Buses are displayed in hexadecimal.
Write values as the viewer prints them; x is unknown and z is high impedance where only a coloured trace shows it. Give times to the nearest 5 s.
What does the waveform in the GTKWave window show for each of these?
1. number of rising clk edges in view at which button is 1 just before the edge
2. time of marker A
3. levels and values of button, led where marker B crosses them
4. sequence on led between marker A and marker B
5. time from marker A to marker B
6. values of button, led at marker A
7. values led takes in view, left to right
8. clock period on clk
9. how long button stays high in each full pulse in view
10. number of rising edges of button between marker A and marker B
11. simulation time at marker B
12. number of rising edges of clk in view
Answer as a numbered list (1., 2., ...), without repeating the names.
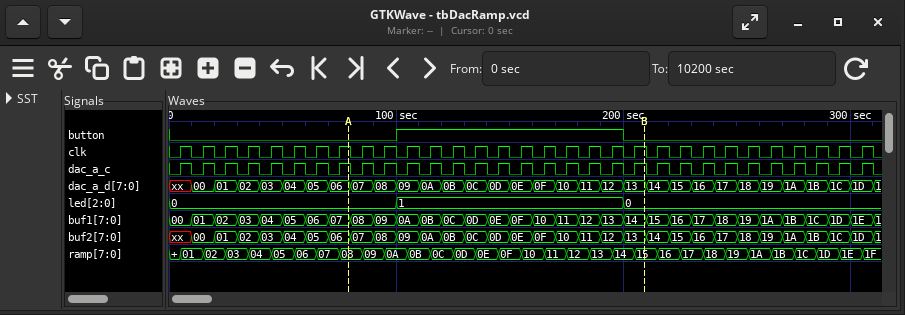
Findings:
1. 10
2. 80 s
3. button=0, led=0
4. 0, 1, 0
5. 130 s
6. button=0, led=0
7. 0, 1, 0
8. 10 s
9. 100 s
10. 1
11. 210 s
12. 31
